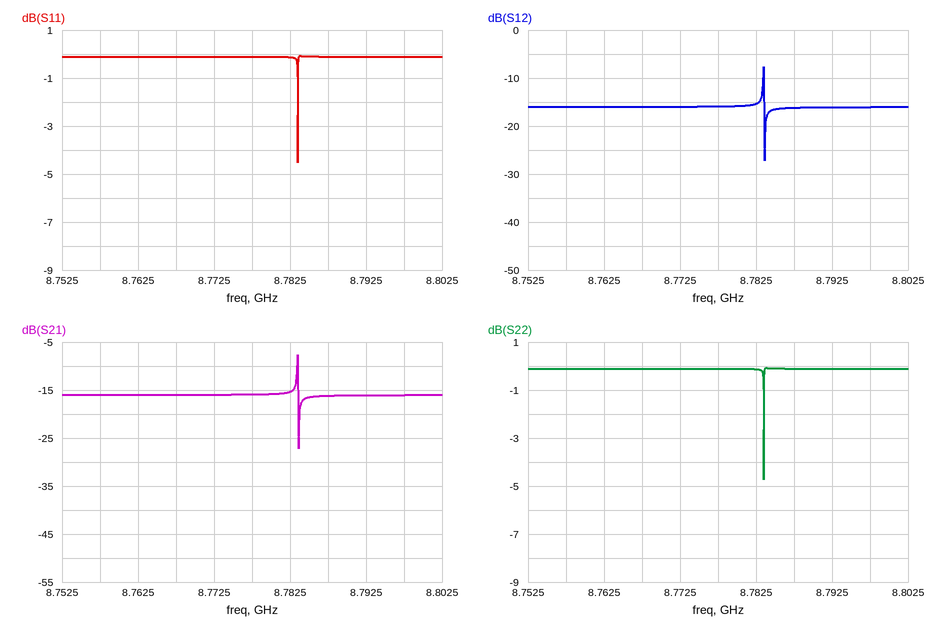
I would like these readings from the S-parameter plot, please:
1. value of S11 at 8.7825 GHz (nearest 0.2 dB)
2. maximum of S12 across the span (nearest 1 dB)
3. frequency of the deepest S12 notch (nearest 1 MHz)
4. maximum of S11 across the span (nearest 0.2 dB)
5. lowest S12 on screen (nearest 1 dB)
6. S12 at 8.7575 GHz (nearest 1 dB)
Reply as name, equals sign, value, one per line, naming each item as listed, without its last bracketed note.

value of S11 at 8.7825 GHz = -0.2 dB
maximum of S12 across the span = -8 dB
frequency of the deepest S12 notch = 8.784 GHz
maximum of S11 across the span = 0.0 dB
lowest S12 on screen = -27 dB
S12 at 8.7575 GHz = -16 dB
